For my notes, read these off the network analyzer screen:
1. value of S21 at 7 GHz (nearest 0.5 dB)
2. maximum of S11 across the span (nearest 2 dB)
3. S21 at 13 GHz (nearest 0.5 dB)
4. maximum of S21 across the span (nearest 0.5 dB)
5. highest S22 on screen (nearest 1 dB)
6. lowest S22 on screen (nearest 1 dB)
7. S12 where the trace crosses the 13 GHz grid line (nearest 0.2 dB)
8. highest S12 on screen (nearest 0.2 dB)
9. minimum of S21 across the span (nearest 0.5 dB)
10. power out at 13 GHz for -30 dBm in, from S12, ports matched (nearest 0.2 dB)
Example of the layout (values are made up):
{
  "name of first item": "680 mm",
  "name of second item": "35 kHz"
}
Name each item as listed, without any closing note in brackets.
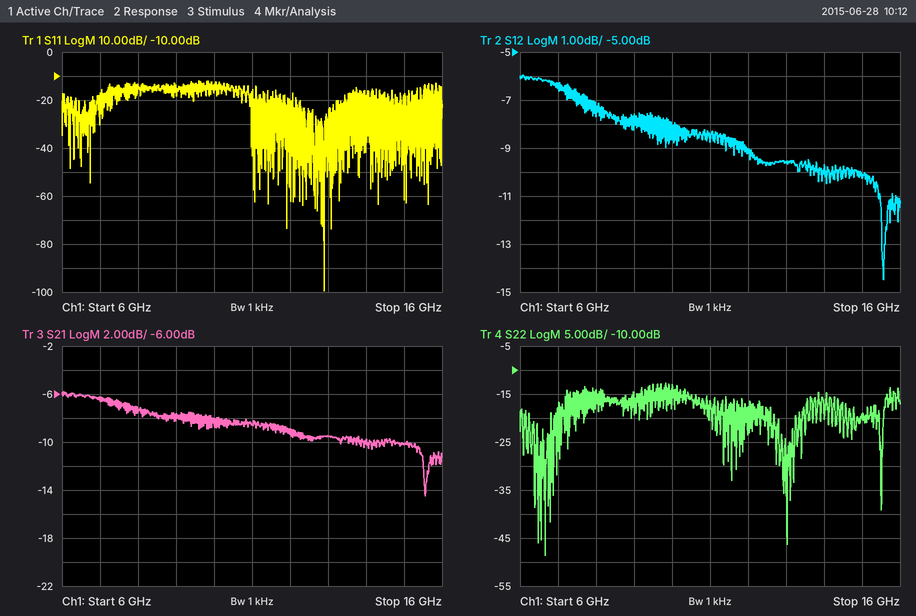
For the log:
{
  "value of S21 at 7 GHz": "-6.5 dB",
  "maximum of S11 across the span": "-12 dB",
  "S21 at 13 GHz": "-9.5 dB",
  "maximum of S21 across the span": "-6.0 dB",
  "highest S22 on screen": "-13 dB",
  "lowest S22 on screen": "-49 dB",
  "S12 where the trace crosses the 13 GHz grid line": "-9.6 dB",
  "highest S12 on screen": "-6.0 dB",
  "minimum of S21 across the span": "-14.5 dB",
  "power out at 13 GHz for -30 dBm in, from S12, ports matched": "-39.6 dBm"
}
